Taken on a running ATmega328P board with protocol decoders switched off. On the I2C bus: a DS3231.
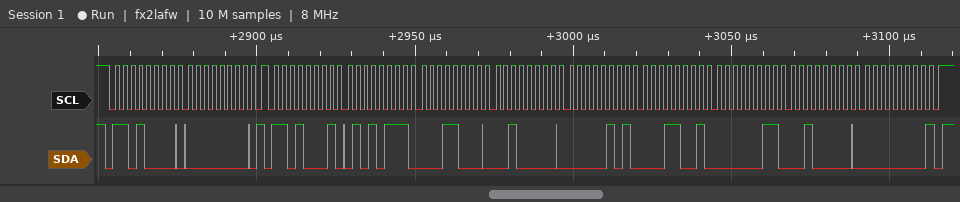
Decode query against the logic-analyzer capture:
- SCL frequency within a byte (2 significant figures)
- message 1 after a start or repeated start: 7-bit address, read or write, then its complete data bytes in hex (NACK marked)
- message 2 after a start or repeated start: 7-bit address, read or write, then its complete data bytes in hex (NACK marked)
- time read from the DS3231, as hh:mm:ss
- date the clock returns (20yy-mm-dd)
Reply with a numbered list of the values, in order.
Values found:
1. 400 kHz
2. 0x68 write: 00
3. 0x68 read: 57 18 20 05 19 03 20 00 NACK
4. 20:18:57
5. 2020-03-19
